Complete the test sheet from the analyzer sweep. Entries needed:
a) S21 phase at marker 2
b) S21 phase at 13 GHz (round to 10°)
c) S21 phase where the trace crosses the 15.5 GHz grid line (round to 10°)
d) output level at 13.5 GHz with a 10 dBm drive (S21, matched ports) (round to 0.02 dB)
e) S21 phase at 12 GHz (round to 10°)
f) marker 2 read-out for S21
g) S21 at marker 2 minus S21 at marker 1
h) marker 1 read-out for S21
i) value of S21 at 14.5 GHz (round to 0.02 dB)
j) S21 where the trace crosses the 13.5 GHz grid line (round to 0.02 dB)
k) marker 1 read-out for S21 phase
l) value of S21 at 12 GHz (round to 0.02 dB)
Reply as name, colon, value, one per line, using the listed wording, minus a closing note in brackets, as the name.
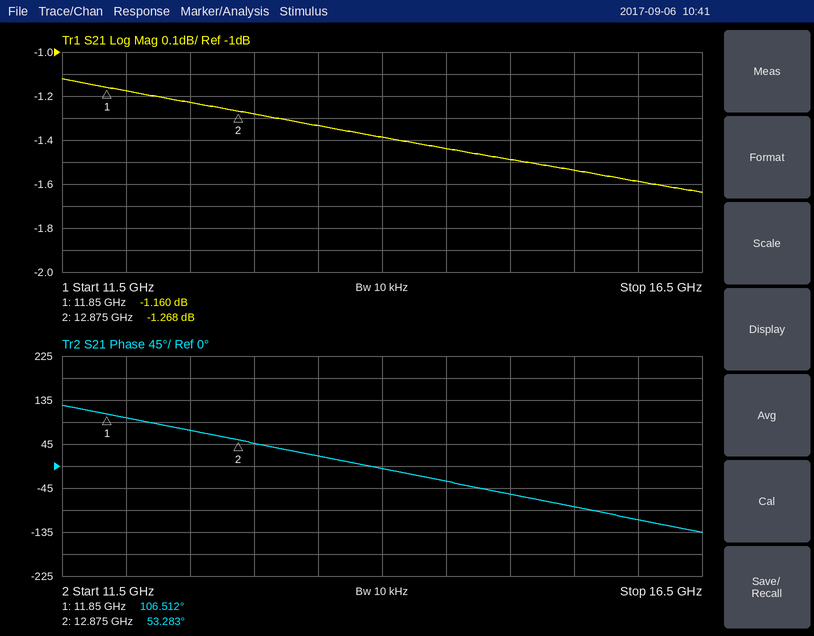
S21 phase at marker 2: 53.283°
S21 phase at 13 GHz: 50°
S21 phase where the trace crosses the 15.5 GHz grid line: -80°
output level at 13.5 GHz with a 10 dBm drive (S21, matched ports): 8.66 dBm
S21 phase at 12 GHz: 100°
marker 2 read-out for S21: -1.268 dB
S21 at marker 2 minus S21 at marker 1: -0.108 dB
marker 1 read-out for S21: -1.160 dB
value of S21 at 14.5 GHz: -1.44 dB
S21 where the trace crosses the 13.5 GHz grid line: -1.34 dB
marker 1 read-out for S21 phase: 106.512°
value of S21 at 12 GHz: -1.18 dB
